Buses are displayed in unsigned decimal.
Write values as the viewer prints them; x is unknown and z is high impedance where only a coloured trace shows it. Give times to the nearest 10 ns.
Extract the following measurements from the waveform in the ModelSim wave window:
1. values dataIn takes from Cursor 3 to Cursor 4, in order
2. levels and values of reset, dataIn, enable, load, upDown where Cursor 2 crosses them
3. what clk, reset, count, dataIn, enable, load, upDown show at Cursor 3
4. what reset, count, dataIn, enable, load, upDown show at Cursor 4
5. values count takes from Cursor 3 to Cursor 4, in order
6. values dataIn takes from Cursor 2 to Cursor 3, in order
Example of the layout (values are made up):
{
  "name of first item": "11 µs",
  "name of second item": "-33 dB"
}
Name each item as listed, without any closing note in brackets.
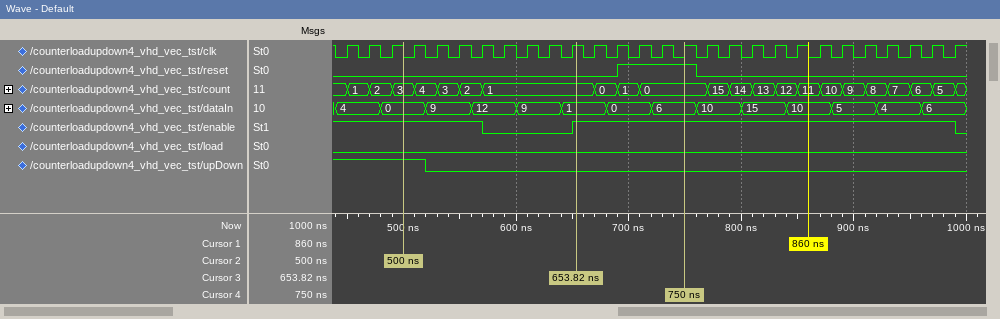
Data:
{
  "values dataIn takes from Cursor 3 to Cursor 4, in order": "1, 0, 6",
  "levels and values of reset, dataIn, enable, load, upDown where Cursor 2 crosses them": "reset=0, dataIn=0, enable=1, load=0, upDown=1",
  "what clk, reset, count, dataIn, enable, load, upDown show at Cursor 3": "clk=1, reset=0, count=1, dataIn=1, enable=1, load=0, upDown=0",
  "what reset, count, dataIn, enable, load, upDown show at Cursor 4": "reset=1, count=0, dataIn=6, enable=1, load=0, upDown=0",
  "values count takes from Cursor 3 to Cursor 4, in order": "1, 0, 1, 0",
  "values dataIn takes from Cursor 2 to Cursor 3, in order": "0, 9, 12, 9, 1"
}
